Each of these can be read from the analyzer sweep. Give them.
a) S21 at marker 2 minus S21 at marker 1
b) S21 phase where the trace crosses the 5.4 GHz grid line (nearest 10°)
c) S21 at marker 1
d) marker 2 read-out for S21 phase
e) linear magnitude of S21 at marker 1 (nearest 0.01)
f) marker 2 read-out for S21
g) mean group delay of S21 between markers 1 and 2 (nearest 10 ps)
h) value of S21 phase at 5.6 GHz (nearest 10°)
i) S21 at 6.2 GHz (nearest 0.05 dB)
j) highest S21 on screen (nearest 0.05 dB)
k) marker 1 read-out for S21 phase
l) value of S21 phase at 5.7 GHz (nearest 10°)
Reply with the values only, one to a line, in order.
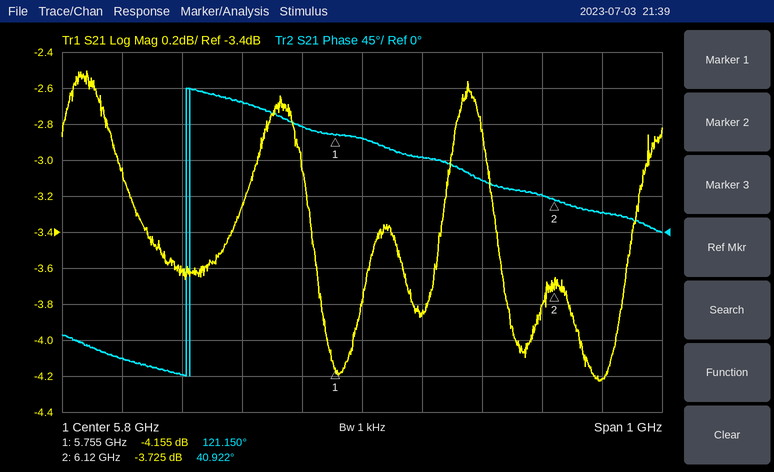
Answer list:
0.430 dB
-160°
-4.155 dB
40.922°
0.62
-3.725 dB
610 ps
160°
-4.20 dB
-2.50 dB
121.150°
130°
